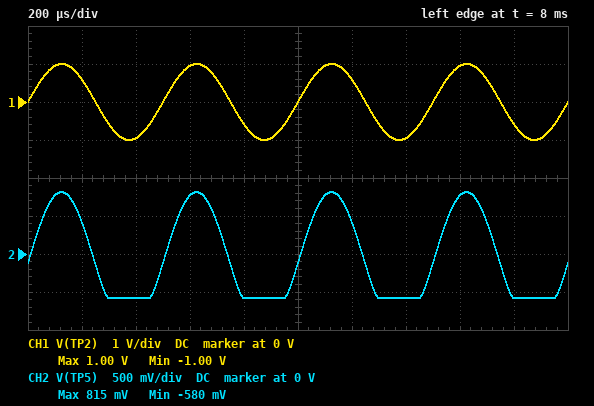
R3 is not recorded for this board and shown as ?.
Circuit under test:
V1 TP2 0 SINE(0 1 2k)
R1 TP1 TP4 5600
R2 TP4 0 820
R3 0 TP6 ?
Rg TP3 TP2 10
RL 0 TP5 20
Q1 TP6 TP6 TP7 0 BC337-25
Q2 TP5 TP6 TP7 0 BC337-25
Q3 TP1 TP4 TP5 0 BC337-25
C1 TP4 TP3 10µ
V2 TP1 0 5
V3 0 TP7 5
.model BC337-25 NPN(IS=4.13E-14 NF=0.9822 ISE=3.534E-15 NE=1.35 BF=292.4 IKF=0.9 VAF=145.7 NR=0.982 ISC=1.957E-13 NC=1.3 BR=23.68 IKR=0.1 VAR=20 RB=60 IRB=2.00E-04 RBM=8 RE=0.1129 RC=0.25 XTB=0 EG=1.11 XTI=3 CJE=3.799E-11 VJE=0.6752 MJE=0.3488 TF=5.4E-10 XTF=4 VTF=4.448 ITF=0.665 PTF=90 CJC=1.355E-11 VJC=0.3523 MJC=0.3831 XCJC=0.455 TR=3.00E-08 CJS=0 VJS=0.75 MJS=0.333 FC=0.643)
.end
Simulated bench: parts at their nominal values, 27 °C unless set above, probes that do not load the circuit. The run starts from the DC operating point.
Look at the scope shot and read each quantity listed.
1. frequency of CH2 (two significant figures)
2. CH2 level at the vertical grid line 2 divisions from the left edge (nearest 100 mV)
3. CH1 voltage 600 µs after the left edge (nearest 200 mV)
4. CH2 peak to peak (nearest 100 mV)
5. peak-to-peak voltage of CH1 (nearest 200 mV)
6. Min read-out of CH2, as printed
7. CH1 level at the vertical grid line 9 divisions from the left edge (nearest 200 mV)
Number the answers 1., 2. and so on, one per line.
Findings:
1. 2.0 kHz
2. -600 mV
3. 1.0 V
4. 1.4 V
5. 2.0 V
6. -580 mV
7. -600 mV
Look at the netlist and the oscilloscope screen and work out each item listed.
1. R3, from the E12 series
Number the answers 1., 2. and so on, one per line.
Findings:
1. 150 Ω
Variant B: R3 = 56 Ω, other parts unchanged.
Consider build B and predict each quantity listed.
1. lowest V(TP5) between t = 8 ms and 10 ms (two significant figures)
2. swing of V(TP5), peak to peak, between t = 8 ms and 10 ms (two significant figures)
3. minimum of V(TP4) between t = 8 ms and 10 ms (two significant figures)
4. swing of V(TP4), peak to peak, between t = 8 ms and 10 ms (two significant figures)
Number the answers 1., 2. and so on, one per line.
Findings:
1. -1.2 V
2. 1.9 V
3. -520 mV
4. 2.0 V
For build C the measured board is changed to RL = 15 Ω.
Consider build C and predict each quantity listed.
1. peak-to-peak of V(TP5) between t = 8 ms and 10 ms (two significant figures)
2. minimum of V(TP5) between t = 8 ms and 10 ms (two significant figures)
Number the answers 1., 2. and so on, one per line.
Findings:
1. 1.2 V
2. -440 mV
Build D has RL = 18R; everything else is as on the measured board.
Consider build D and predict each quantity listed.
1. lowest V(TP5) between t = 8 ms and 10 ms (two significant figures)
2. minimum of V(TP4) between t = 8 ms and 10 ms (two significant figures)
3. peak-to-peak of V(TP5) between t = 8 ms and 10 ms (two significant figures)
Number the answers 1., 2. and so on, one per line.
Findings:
1. -520 mV
2. -420 mV
3. 1.3 V
